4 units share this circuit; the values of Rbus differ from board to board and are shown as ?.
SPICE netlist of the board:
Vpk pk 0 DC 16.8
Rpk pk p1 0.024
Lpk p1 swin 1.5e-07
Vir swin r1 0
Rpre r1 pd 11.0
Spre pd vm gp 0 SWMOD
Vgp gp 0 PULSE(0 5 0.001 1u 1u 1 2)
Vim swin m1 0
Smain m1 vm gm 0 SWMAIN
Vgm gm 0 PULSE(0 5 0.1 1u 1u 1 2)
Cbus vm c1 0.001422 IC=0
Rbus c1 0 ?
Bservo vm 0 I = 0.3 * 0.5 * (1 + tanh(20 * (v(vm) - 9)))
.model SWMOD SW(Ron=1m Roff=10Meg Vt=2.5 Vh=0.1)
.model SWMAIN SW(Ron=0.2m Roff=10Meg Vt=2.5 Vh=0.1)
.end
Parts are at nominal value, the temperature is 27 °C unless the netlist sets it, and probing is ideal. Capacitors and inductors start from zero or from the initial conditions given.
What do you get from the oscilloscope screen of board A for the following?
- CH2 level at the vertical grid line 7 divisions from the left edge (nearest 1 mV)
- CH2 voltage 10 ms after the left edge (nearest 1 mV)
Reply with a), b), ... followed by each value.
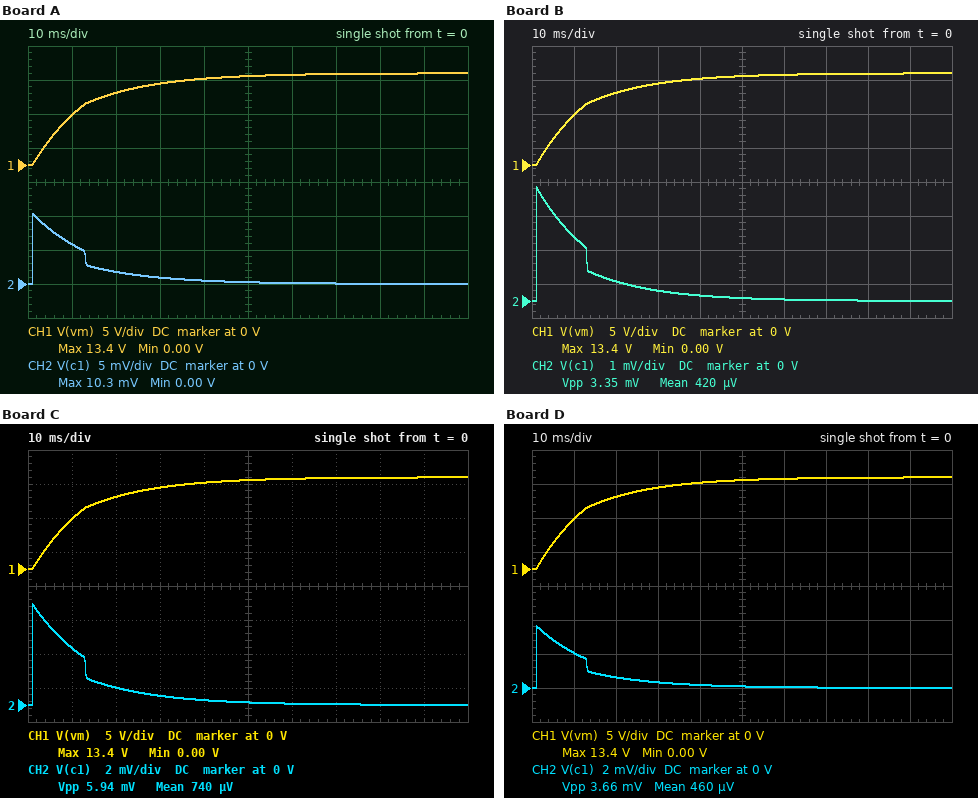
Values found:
a) 0 V
b) 6 mV
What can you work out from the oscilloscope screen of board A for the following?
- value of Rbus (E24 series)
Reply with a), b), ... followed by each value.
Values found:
a) 6.8 mΩ
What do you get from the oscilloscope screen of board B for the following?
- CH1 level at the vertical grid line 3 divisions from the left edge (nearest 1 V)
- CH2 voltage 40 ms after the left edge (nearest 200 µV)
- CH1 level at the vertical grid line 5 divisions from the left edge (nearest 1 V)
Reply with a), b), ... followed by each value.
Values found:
a) 12 V
b) 200 µV
c) 13 V
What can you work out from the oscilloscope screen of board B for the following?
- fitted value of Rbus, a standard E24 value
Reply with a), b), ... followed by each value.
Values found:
a) 2.2 mΩ
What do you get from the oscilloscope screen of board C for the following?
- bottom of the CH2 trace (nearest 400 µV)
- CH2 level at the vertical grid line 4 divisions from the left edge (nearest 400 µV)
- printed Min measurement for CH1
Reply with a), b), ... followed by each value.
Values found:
a) 0 V
b) 400 µV
c) 0.00 V
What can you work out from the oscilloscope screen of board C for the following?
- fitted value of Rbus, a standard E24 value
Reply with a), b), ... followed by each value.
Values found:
a) 3.9 mΩ
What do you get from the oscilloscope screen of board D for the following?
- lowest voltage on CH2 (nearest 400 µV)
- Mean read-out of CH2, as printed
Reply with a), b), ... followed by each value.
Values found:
a) 0 V
b) 460 µV
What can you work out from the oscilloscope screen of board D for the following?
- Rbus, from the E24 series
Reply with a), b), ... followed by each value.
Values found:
a) 2.4 mΩ
